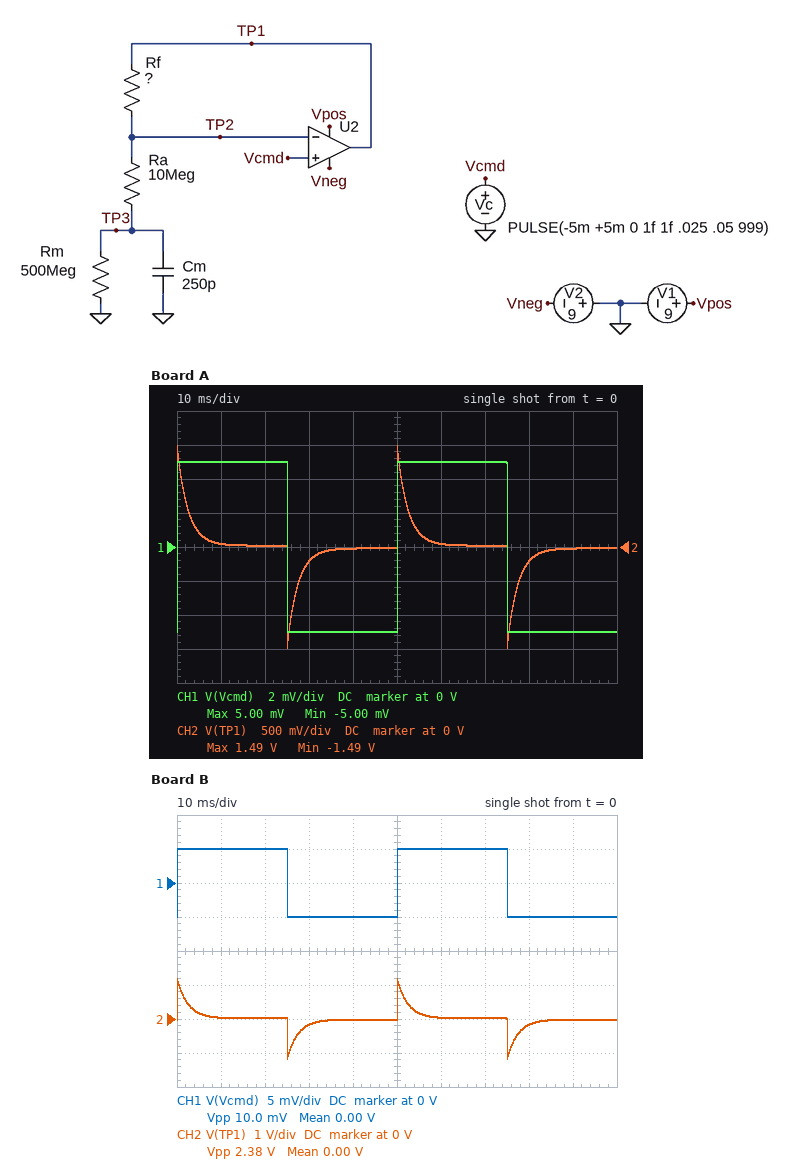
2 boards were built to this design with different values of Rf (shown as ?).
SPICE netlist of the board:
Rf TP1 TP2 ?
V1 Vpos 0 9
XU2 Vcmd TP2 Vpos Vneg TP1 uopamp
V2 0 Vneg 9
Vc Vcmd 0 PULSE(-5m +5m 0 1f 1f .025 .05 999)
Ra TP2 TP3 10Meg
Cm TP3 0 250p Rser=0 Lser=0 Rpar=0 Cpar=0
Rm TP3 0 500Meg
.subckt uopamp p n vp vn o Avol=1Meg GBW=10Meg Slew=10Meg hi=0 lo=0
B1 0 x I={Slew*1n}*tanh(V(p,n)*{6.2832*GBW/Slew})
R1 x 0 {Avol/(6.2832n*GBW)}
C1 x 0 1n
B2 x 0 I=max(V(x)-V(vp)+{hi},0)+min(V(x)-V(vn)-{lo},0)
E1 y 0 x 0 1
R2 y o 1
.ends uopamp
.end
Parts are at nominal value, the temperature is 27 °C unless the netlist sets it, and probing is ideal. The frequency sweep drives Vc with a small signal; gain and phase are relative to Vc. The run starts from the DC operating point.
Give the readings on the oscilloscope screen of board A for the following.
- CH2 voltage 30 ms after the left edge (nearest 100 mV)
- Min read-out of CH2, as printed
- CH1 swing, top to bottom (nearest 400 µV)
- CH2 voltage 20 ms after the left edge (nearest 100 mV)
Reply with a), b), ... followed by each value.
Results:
a) -200 mV
b) -1.49 V
c) 10.0 mV
d) 0 V
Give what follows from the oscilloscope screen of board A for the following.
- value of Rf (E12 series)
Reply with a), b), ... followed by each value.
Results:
a) 1.5 GΩ
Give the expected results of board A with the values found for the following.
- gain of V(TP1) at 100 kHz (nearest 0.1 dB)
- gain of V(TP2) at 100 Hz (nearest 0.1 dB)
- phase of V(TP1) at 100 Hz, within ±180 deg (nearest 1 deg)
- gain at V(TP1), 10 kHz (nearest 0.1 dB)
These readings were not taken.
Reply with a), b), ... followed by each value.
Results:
a) 38.4 dB
b) 0 dB
c) 32 deg
d) 43.5 dB
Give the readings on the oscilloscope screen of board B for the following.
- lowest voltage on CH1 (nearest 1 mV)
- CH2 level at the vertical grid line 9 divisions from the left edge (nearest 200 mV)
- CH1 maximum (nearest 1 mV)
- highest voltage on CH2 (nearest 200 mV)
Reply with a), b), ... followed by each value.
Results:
a) -5 mV
b) 0 V
c) 5 mV
d) 1.2 V
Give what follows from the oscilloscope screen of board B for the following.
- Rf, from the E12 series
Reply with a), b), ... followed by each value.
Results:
a) 1.2 GΩ
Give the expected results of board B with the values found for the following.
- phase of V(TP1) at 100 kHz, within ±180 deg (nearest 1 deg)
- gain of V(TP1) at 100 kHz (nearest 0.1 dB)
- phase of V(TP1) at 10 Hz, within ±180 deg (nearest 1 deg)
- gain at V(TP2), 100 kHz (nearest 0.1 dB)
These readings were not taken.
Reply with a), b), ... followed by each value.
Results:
a) -50 deg
b) 37.7 dB
c) 71 deg
d) -3.9 dB
